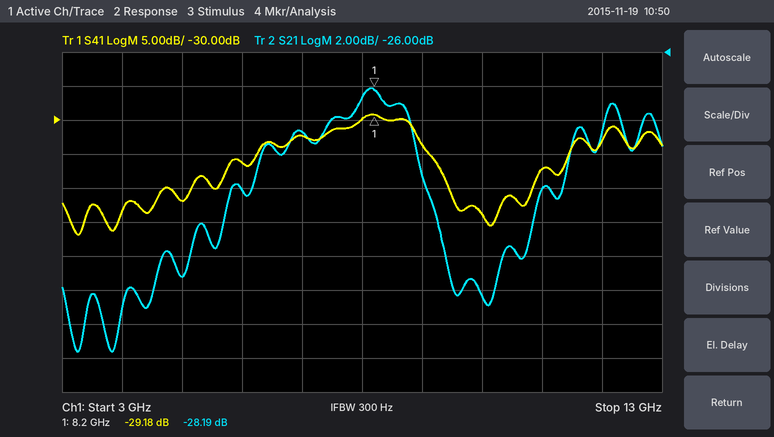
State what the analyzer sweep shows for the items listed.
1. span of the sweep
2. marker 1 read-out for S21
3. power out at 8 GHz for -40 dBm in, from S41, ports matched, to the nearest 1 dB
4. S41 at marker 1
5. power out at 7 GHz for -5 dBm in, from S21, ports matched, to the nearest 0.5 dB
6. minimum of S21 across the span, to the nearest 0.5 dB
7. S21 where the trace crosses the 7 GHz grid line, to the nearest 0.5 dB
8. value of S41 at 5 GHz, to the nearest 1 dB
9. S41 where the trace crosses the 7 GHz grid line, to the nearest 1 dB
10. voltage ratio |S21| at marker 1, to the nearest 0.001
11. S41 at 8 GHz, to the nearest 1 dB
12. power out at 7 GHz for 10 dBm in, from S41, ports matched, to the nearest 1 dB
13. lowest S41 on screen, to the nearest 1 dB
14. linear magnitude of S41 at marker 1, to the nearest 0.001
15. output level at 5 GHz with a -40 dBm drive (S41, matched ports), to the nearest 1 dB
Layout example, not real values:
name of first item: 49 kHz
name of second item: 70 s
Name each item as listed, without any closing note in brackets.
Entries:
span of the sweep: 10 GHz
marker 1 read-out for S21: -28.19 dB
power out at 8 GHz for -40 dBm in, from S41, ports matched, to the nearest 1 dB: -70 dBm
S41 at marker 1: -29.18 dB
power out at 7 GHz for -5 dBm in, from S21, ports matched, to the nearest 0.5 dB: -35.5 dBm
minimum of S21 across the span, to the nearest 0.5 dB: -43.5 dB
S21 where the trace crosses the 7 GHz grid line, to the nearest 0.5 dB: -30.5 dB
value of S41 at 5 GHz, to the nearest 1 dB: -42 dB
S41 where the trace crosses the 7 GHz grid line, to the nearest 1 dB: -32 dB
voltage ratio |S21| at marker 1, to the nearest 0.001: 0.039
S41 at 8 GHz, to the nearest 1 dB: -30 dB
power out at 7 GHz for 10 dBm in, from S41, ports matched, to the nearest 1 dB: -22 dBm
lowest S41 on screen, to the nearest 1 dB: -47 dB
linear magnitude of S41 at marker 1, to the nearest 0.001: 0.035
output level at 5 GHz with a -40 dBm drive (S41, matched ports), to the nearest 1 dB: -82 dBm
